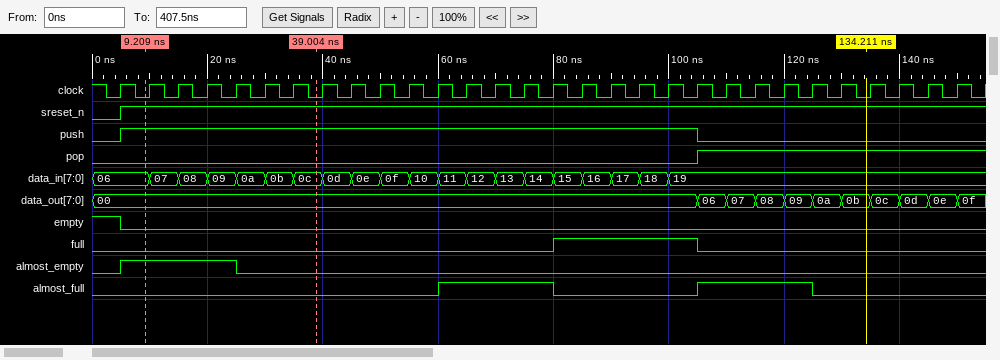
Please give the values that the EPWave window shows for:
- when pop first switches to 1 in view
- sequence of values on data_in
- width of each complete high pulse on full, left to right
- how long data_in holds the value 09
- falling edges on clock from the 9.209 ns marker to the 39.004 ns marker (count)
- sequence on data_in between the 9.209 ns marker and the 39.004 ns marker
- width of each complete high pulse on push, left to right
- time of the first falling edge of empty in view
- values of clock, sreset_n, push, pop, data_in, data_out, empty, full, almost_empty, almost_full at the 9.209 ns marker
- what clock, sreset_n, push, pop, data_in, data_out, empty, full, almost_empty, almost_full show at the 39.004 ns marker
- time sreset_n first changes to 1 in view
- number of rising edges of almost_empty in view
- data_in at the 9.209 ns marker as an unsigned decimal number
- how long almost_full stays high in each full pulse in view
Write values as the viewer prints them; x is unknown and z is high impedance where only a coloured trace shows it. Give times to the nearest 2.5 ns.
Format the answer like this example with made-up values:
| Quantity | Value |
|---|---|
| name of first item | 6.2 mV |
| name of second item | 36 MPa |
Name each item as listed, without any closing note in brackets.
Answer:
| Quantity | Value |
|---|---|
| when pop first switches to 1 in view | 105 ns |
| sequence of values on data_in | 06, 07, 08, 09, 0a, 0b, 0c, 0d, 0e, 0f, 10, 11, 12, 13, 14, 15, 16, 17, 18, 19 |
| width of each complete high pulse on full, left to right | 25 ns |
| how long data_in holds the value 09 | 5 ns |
| falling edges on clock from the 9.209 ns marker to the 39.004 ns marker | 6 |
| sequence on data_in between the 9.209 ns marker and the 39.004 ns marker | 06, 07, 08, 09, 0a, 0b, 0c |
| width of each complete high pulse on push, left to right | 100 ns |
| time of the first falling edge of empty in view | 5 ns |
| values of clock, sreset_n, push, pop, data_in, data_out, empty, full, almost_empty, almost_full at the 9.209 ns marker | clock=0, sreset_n=1, push=1, pop=0, data_in=06, data_out=00, empty=0, full=0, almost_empty=1, almost_full=0 |
| what clock, sreset_n, push, pop, data_in, data_out, empty, full, almost_empty, almost_full show at the 39.004 ns marker | clock=0, sreset_n=1, push=1, pop=0, data_in=0c, data_out=00, empty=0, full=0, almost_empty=0, almost_full=0 |
| time sreset_n first changes to 1 in view | 5 ns |
| number of rising edges of almost_empty in view | 1 |
| data_in at the 9.209 ns marker as an unsigned decimal number | 6 |
| how long almost_full stays high in each full pulse in view | 20 ns, 20 ns |
